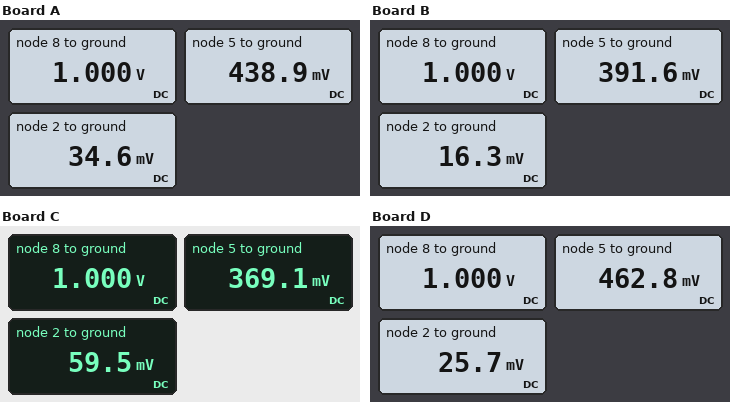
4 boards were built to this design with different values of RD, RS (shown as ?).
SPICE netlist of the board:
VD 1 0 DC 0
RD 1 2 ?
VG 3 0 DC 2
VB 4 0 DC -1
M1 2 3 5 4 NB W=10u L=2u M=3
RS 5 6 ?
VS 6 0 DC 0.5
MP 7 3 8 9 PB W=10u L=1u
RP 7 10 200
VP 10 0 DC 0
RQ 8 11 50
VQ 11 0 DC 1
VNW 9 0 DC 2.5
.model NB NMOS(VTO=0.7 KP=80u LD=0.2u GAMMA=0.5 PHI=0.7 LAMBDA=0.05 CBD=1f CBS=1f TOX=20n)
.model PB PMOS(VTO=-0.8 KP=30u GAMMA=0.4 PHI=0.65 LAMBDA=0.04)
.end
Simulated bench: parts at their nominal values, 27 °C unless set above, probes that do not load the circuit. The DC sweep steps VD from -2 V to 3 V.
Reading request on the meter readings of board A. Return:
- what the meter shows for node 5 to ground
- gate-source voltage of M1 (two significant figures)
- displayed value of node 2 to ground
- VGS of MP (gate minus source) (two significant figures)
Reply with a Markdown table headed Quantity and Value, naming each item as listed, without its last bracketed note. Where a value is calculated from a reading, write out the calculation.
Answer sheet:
| Quantity | Value |
|---|---|
| what the meter shows for node 5 to ground | 438.9 mV |
| gate-source voltage of M1 | 2 V - 438.9 mV = 1.6 V |
| displayed value of node 2 to ground | 34.6 mV |
| VGS of MP (gate minus source) | 2 V - 1 V = 1.0 V |
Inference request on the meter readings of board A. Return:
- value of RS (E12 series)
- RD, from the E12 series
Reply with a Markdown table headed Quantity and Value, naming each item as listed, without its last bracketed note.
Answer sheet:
| Quantity | Value |
|---|---|
| value of RS | 120 Ω |
| RD, from the E12 series | 68 Ω |
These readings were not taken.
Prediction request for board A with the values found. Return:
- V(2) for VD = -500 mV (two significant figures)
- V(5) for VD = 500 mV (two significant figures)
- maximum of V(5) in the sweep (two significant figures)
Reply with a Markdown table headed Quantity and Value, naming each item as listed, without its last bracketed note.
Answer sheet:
| Quantity | Value |
|---|---|
| V(2) for VD = -500 mV | -410 mV |
| V(5) for VD = 500 mV | 500 mV |
| maximum of V(5) in the sweep | 520 mV |
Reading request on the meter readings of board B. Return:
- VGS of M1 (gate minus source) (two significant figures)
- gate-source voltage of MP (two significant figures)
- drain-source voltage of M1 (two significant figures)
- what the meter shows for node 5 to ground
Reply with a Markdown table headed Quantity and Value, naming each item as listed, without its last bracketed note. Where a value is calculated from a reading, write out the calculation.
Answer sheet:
| Quantity | Value |
|---|---|
| VGS of M1 (gate minus source) | 2 V - 391.6 mV = 1.6 V |
| gate-source voltage of MP | 2 V - 1 V = 1.0 V |
| drain-source voltage of M1 | 16.3 mV - 391.6 mV = -380 mV |
| what the meter shows for node 5 to ground | 391.6 mV |
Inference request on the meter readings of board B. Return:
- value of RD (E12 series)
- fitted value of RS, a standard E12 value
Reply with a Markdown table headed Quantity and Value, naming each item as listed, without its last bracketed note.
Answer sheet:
| Quantity | Value |
|---|---|
| value of RD | 33 Ω |
| fitted value of RS, a standard E12 value | 220 Ω |
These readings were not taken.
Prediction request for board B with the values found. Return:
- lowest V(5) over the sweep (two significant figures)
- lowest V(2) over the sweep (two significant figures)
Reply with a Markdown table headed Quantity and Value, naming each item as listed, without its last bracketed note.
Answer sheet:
| Quantity | Value |
|---|---|
| lowest V(5) over the sweep | -530 mV |
| lowest V(2) over the sweep | -1.7 V |
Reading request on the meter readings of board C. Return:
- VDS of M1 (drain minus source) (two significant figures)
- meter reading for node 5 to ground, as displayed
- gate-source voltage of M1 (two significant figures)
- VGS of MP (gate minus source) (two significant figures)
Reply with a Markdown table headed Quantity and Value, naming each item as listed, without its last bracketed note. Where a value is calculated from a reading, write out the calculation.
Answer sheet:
| Quantity | Value |
|---|---|
| VDS of M1 (drain minus source) | 59.5 mV - 369.1 mV = -310 mV |
| meter reading for node 5 to ground, as displayed | 369.1 mV |
| gate-source voltage of M1 | 2 V - 369.1 mV = 1.6 V |
| VGS of MP (gate minus source) | 2 V - 1 V = 1.0 V |
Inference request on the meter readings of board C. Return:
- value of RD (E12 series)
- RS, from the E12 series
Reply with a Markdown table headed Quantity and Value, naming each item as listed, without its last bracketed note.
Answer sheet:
| Quantity | Value |
|---|---|
| value of RD | 150 Ω |
| RS, from the E12 series | 330 Ω |
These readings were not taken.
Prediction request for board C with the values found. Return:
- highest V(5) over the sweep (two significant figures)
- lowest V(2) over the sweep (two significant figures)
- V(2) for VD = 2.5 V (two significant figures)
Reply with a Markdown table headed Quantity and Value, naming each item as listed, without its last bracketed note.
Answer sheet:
| Quantity | Value |
|---|---|
| highest V(5) over the sweep | 550 mV |
| lowest V(2) over the sweep | -1.5 V |
| V(2) for VD = 2.5 V | 2.5 V |
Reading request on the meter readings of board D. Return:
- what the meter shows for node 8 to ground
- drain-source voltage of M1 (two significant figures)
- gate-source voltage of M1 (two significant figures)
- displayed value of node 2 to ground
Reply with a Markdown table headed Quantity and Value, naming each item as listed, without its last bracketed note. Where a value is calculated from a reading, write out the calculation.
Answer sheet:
| Quantity | Value |
|---|---|
| what the meter shows for node 8 to ground | 1.000 V |
| drain-source voltage of M1 | 25.7 mV - 462.8 mV = -440 mV |
| gate-source voltage of M1 | 2 V - 462.8 mV = 1.5 V |
| displayed value of node 2 to ground | 25.7 mV |
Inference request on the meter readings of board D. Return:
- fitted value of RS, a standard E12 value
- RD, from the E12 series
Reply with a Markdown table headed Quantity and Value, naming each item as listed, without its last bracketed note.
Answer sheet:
| Quantity | Value |
|---|---|
| fitted value of RS, a standard E12 value | 68 Ω |
| RD, from the E12 series | 47 Ω |
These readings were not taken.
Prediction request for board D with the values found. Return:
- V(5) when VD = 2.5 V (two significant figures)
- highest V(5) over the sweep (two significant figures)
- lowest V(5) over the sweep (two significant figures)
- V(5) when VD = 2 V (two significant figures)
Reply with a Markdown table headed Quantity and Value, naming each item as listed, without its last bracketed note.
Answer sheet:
| Quantity | Value |
|---|---|
| V(5) when VD = 2.5 V | 510 mV |
| highest V(5) over the sweep | 510 mV |
| lowest V(5) over the sweep | 71 mV |
| V(5) when VD = 2 V | 510 mV |
